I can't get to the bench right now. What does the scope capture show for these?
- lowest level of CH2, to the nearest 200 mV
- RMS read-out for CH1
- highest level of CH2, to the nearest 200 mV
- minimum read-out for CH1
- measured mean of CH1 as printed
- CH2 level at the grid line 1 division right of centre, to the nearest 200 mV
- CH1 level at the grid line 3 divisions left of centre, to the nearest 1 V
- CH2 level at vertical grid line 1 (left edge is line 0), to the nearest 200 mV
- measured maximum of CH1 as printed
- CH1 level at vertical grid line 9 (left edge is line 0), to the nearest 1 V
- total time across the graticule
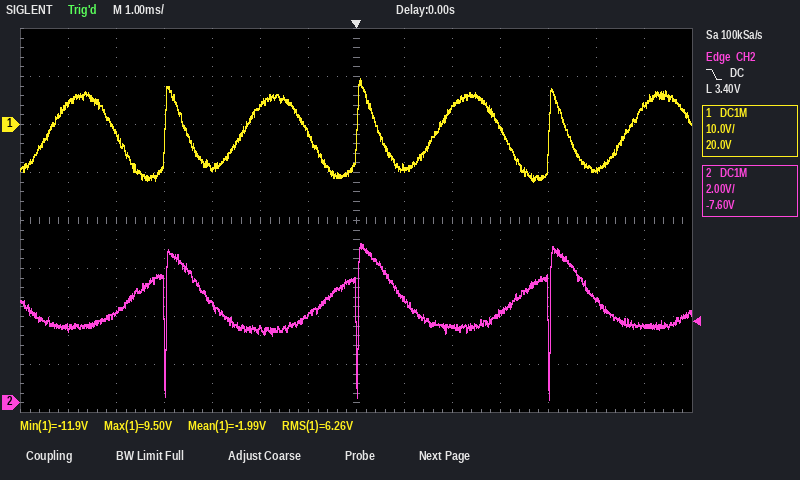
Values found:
200 mV
6.26 V
6.6 V
-11.9 V
-1.99 V
4.4 V
-9 V
3.2 V
9.50 V
4 V
14 ms
